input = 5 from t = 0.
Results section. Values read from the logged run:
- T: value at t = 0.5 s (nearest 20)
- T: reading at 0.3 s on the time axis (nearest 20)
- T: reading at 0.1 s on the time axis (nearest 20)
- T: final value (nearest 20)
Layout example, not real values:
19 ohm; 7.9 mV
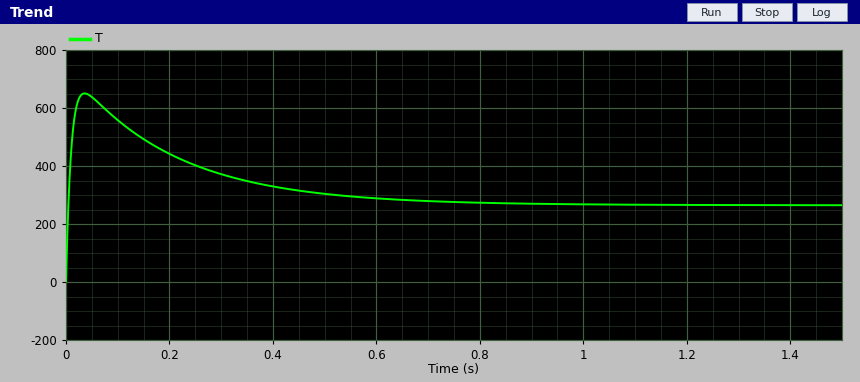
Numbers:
300; 380; 560; 260
